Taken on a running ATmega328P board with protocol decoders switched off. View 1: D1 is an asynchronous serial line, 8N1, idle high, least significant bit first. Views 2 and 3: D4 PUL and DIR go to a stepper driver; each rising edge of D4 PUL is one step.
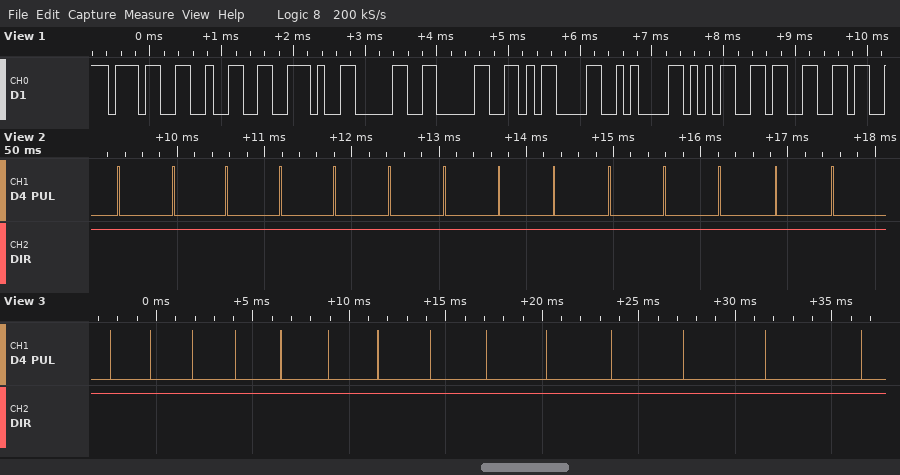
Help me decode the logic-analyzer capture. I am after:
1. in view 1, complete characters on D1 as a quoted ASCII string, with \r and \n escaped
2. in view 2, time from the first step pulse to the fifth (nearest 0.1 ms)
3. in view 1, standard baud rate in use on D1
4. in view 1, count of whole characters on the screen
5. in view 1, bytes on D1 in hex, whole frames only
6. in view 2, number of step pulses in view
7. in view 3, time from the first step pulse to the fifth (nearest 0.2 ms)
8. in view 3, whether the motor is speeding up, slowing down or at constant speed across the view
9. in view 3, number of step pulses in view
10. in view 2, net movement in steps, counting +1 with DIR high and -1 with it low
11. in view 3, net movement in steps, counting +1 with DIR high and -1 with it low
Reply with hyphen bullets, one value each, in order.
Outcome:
- "72.00\r\n53"
- 2.5 ms
- 9600 baud
- 9
- 0x37 0x32 0x2E 0x30 0x30 0x0D 0x0A 0x35 0x33
- 14
- 8.8 ms
- slowing down
- 14
- +14
- +14
